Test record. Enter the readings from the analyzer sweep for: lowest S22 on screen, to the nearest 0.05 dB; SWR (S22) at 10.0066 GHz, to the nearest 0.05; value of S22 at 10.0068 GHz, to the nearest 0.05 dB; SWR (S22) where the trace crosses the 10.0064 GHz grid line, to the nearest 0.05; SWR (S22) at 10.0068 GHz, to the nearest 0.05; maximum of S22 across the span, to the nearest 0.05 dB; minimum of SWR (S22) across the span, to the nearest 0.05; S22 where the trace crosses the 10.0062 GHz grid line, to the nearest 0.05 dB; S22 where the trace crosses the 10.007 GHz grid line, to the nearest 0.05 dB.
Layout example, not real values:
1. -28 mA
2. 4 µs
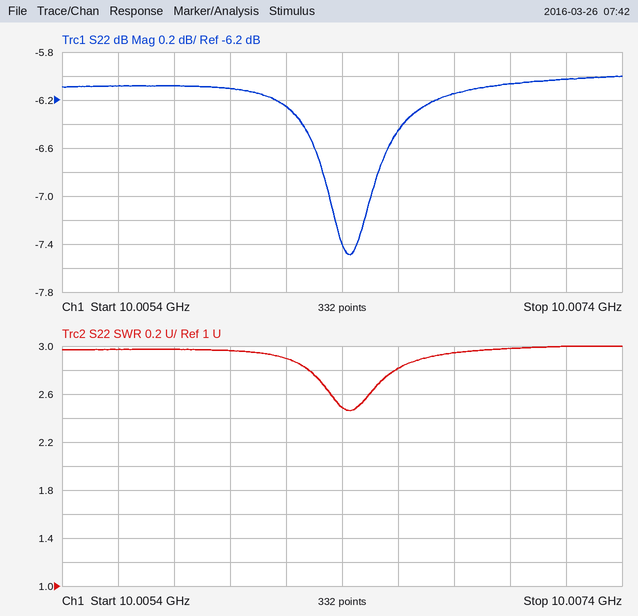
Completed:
1. -7.50 dB
2. 2.80
3. -6.15 dB
4. 2.50
5. 2.95
6. -6.00 dB
7. 2.45
8. -6.25 dB
9. -6.05 dB
